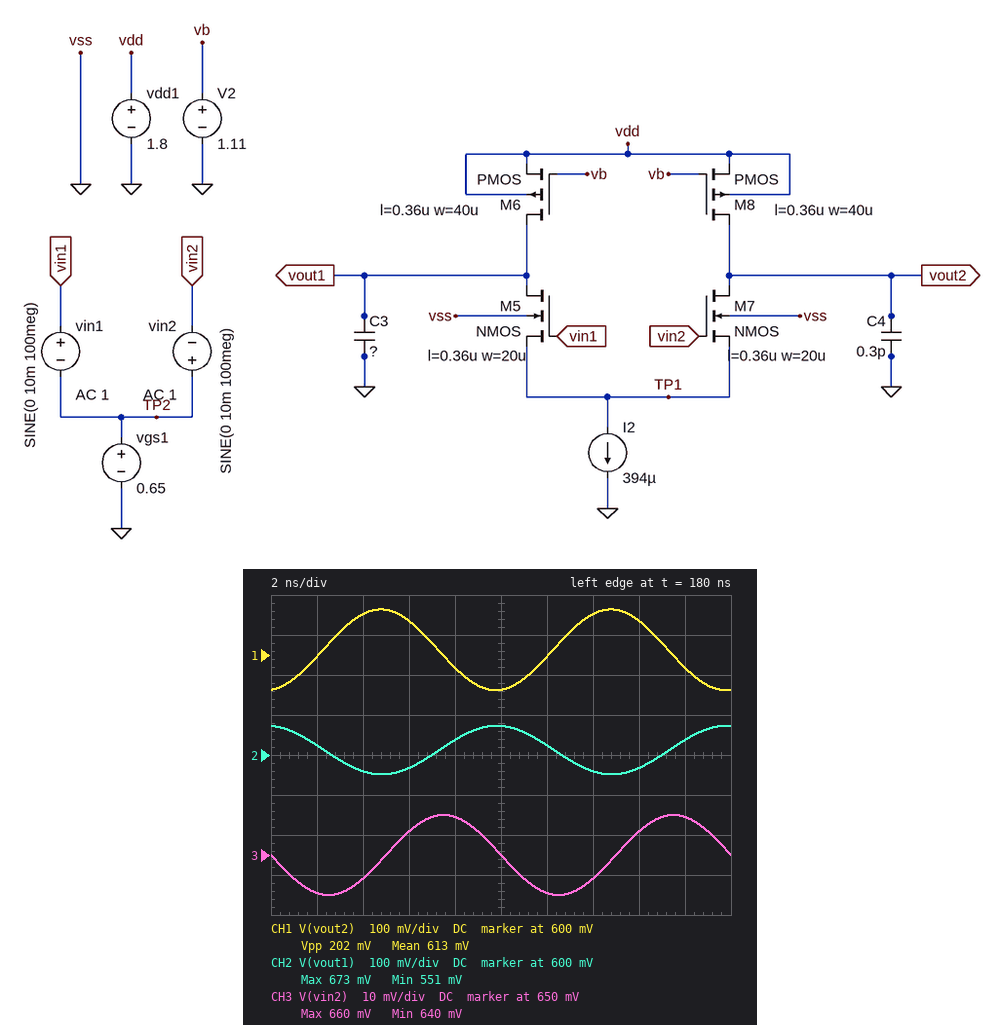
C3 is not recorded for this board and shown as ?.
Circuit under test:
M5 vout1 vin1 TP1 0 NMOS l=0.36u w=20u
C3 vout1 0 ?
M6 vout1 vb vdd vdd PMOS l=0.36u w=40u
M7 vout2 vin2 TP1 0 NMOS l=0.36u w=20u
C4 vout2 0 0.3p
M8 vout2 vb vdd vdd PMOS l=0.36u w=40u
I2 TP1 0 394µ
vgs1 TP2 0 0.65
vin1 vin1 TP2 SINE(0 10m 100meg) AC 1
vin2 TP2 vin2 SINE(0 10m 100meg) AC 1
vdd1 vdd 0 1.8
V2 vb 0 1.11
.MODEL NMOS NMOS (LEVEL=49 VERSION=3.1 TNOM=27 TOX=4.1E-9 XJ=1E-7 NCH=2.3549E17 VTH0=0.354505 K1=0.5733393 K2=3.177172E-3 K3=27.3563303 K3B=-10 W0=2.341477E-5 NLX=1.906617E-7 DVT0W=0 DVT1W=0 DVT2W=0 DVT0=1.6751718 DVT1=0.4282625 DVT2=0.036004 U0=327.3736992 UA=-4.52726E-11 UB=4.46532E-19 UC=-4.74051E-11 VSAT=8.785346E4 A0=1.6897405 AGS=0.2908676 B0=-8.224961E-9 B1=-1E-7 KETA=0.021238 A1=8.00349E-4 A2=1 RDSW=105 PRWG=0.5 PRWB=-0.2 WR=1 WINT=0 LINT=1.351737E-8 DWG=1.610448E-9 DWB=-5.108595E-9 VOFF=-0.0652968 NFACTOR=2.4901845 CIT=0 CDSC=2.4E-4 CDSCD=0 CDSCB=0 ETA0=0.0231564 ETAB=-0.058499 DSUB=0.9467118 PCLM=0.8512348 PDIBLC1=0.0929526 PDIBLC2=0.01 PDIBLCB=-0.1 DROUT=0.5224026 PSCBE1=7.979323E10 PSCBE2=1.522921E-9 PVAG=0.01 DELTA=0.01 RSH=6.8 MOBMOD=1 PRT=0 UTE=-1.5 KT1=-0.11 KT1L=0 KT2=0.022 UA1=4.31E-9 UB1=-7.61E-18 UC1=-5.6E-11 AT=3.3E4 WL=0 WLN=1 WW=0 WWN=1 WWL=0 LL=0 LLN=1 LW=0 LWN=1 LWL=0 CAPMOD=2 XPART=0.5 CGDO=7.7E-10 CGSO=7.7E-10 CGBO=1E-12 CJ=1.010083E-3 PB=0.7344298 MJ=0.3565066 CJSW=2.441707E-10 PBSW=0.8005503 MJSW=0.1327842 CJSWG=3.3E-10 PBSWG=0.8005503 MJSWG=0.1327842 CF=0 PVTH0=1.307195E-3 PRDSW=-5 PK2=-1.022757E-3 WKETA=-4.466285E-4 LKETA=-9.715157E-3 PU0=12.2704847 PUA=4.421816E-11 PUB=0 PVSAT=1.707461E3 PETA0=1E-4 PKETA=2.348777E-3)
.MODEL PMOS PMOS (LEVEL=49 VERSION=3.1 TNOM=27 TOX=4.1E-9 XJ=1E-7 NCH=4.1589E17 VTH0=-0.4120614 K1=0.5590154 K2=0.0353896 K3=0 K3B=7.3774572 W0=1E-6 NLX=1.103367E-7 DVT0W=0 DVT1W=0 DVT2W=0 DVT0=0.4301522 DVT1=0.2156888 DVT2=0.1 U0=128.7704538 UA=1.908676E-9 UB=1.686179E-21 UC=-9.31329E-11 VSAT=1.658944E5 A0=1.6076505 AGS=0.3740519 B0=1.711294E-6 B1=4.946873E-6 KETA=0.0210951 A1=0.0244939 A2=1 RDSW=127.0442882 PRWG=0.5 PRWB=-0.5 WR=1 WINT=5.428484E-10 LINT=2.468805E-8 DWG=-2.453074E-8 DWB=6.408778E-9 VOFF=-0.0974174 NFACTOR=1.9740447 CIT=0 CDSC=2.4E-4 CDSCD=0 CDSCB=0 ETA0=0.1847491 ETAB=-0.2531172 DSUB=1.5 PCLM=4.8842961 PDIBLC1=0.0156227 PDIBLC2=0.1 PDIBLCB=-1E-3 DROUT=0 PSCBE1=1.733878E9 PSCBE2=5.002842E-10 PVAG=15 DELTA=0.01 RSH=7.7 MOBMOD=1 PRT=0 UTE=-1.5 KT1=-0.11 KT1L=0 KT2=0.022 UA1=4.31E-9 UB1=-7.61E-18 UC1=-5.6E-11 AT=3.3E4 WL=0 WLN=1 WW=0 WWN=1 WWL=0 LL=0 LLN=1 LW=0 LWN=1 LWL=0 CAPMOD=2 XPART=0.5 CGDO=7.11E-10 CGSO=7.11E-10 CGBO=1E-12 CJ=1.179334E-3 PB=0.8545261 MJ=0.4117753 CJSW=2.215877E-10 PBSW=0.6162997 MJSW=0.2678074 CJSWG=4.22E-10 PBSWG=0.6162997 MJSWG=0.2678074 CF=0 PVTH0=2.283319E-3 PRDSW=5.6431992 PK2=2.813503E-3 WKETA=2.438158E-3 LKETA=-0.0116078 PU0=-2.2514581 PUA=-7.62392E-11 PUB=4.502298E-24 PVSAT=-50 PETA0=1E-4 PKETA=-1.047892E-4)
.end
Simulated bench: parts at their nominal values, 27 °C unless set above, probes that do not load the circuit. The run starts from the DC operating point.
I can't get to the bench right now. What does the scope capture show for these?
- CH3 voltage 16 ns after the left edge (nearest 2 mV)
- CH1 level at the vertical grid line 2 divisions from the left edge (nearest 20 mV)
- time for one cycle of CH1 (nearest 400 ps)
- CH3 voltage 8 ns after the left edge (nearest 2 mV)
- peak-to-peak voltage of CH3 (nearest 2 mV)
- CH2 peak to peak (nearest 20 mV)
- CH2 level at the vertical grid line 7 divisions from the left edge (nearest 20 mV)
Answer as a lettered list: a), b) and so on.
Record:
a) 656 mV
b) 700 mV
c) 10.0 ns
d) 660 mV
e) 20 mV
f) 120 mV
g) 560 mV
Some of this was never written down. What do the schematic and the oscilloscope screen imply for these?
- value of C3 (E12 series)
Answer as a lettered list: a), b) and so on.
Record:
a) 560 fF
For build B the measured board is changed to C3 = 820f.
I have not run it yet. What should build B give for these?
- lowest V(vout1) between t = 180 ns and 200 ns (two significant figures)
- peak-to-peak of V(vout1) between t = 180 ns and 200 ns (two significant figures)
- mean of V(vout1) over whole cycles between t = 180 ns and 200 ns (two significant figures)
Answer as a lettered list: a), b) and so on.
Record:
a) 570 mV
b) 85 mV
c) 610 mV
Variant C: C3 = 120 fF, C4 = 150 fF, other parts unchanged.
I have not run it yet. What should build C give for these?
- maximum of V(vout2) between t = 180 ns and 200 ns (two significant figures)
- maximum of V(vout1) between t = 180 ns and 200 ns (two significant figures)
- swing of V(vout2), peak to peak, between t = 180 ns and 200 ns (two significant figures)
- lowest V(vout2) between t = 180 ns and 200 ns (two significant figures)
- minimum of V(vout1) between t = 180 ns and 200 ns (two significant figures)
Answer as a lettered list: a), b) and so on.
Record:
a) 780 mV
b) 830 mV
c) 330 mV
d) 450 mV
e) 400 mV
